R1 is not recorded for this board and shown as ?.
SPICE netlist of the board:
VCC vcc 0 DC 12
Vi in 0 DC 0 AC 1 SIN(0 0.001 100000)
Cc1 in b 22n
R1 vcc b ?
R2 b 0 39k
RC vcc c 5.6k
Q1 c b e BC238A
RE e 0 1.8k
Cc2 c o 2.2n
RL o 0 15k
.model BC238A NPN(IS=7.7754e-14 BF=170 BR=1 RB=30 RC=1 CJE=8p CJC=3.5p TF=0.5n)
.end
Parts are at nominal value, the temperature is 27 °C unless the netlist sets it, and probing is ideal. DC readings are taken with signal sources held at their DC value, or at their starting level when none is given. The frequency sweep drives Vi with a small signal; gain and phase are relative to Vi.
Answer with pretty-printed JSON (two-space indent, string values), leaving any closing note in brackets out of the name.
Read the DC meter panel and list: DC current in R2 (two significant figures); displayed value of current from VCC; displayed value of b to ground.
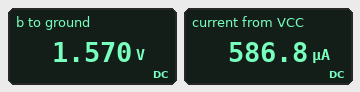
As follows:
{
  "DC current in R2": "40 µA",
  "displayed value of current from VCC": "586.8 µA",
  "displayed value of b to ground": "1.570 V"
}
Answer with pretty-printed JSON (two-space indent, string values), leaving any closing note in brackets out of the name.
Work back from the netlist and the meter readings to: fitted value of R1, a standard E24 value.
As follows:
{
  "fitted value of R1, a standard E24 value": "240 kΩ"
}
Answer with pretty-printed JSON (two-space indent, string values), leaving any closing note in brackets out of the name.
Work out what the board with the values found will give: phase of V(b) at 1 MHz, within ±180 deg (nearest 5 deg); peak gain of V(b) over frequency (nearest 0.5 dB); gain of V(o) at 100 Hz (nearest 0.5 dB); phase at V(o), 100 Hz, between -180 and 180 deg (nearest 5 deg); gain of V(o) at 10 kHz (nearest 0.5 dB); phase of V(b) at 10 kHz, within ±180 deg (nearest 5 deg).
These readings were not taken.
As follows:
{
  "phase of V(b) at 1 MHz, within ±180 deg": "0 deg",
  "peak gain of V(b) over frequency": "0 dB",
  "gain of V(o) at 100 Hz": "-32.5 dB",
  "phase at V(o), 100 Hz, between -180 and 180 deg": "-25 deg",
  "gain of V(o) at 10 kHz": "6.5 dB",
  "phase of V(b) at 10 kHz, within ±180 deg": "0 deg"
}
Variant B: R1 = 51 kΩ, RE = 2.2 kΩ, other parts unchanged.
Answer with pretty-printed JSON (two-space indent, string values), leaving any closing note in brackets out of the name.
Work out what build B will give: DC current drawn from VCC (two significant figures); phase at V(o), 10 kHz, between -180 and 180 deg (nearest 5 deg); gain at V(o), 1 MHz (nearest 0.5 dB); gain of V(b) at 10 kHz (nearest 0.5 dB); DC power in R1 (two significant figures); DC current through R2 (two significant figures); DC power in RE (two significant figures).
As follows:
{
  "DC current drawn from VCC": "1.7 mA",
  "phase at V(o), 10 kHz, between -180 and 180 deg": "50 deg",
  "gain at V(o), 1 MHz": "-4.0 dB",
  "gain of V(b) at 10 kHz": "-1.0 dB",
  "DC power in R1": "1.2 mW",
  "DC current through R2": "100 µA",
  "DC power in RE": "5.4 mW"
}
